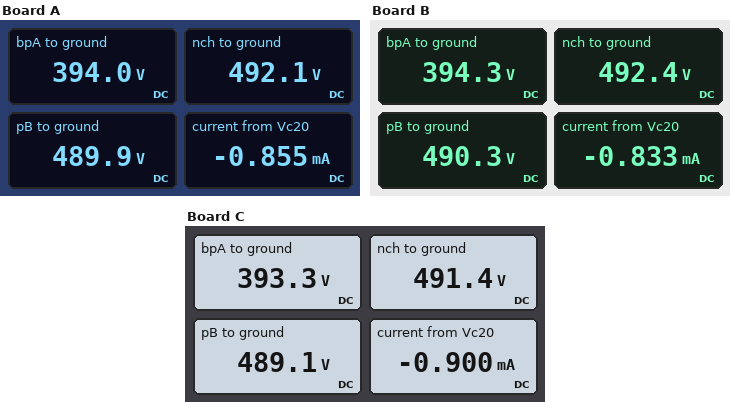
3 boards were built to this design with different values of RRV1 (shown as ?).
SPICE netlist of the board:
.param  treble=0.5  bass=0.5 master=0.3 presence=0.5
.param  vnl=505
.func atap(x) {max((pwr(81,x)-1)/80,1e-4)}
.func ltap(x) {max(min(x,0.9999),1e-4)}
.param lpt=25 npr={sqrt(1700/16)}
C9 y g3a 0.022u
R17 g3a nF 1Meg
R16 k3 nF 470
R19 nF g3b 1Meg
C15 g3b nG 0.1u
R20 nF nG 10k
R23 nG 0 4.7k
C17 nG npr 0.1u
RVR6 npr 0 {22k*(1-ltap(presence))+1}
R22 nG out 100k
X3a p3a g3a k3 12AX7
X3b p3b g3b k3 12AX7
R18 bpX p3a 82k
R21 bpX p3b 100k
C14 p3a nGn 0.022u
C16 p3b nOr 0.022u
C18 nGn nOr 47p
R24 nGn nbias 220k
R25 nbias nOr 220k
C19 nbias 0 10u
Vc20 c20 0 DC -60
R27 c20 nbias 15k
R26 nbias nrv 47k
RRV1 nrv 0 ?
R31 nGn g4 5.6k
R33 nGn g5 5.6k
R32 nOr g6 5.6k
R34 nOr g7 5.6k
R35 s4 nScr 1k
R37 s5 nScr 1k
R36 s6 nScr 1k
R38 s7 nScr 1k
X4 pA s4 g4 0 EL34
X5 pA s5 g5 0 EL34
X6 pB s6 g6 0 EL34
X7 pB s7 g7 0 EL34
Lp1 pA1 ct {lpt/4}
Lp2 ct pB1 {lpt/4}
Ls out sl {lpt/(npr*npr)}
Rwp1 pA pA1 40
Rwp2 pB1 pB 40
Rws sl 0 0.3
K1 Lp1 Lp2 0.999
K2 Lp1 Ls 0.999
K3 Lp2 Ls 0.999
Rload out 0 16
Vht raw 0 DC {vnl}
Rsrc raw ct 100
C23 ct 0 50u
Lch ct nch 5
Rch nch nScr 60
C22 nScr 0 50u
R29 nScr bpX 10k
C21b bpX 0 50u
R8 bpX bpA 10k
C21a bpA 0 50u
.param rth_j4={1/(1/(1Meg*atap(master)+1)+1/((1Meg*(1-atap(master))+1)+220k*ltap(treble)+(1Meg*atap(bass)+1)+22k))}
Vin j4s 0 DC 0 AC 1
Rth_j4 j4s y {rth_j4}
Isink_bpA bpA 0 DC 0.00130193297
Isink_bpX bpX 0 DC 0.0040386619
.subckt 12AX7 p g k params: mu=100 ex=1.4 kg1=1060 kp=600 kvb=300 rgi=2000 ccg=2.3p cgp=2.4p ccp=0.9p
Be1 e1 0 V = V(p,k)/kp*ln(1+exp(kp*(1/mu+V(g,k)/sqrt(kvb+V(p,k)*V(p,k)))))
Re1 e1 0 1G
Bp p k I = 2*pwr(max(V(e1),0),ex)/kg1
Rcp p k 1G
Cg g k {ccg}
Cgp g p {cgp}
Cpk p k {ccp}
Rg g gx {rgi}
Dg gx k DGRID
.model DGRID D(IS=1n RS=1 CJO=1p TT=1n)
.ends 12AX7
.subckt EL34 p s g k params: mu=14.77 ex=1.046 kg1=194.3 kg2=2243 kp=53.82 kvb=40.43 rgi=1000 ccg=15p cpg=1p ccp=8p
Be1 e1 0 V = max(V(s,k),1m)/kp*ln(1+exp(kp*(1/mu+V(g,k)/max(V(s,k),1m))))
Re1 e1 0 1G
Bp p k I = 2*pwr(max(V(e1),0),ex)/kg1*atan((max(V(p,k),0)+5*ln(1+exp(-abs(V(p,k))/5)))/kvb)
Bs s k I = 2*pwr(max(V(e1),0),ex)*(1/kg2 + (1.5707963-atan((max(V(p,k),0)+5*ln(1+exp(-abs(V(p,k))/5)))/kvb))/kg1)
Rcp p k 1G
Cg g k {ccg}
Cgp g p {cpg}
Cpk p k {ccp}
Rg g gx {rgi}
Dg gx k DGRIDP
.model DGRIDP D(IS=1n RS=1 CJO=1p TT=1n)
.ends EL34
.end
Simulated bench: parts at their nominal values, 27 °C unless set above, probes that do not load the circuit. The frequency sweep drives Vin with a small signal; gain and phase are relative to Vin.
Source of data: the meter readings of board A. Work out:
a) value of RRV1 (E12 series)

8.2 kΩ
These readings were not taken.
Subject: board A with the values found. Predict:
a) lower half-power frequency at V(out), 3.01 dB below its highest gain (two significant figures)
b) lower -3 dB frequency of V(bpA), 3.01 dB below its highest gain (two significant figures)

19 Hz
74 mHz
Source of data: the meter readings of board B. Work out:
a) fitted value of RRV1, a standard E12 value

10 kΩ
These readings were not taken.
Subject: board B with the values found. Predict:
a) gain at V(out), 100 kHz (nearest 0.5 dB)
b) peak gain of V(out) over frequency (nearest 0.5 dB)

17.0 dB
22.0 dB
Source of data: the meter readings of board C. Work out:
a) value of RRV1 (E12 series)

4.7 kΩ
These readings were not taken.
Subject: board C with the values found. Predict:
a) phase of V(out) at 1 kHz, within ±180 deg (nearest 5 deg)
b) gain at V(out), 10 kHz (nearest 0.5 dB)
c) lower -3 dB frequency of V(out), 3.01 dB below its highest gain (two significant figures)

0 deg
22.5 dB
18 Hz
